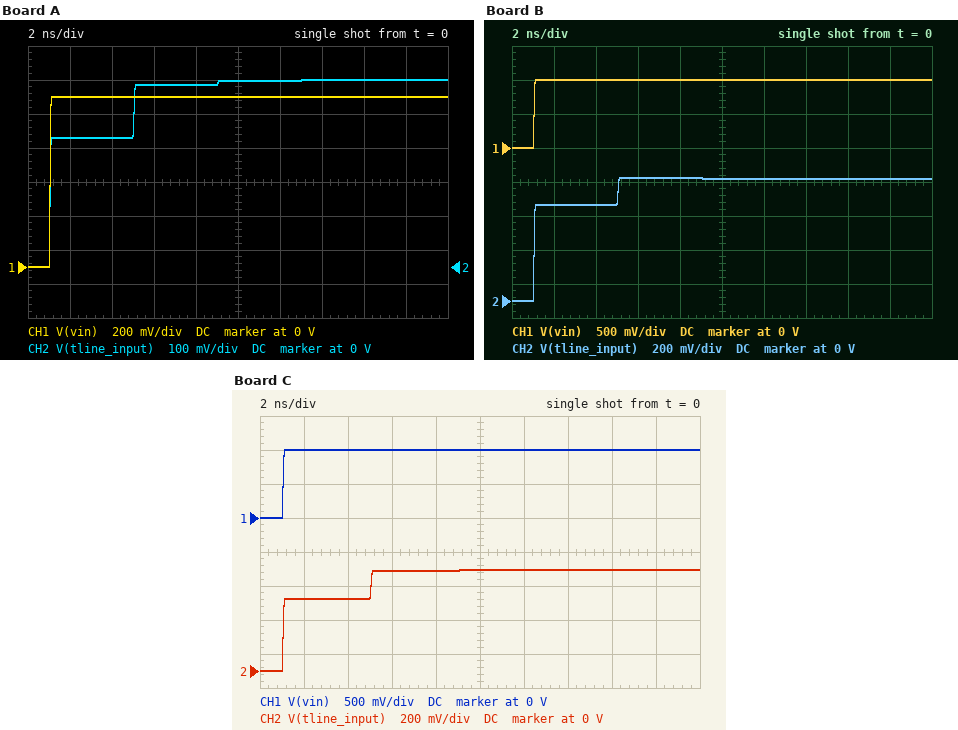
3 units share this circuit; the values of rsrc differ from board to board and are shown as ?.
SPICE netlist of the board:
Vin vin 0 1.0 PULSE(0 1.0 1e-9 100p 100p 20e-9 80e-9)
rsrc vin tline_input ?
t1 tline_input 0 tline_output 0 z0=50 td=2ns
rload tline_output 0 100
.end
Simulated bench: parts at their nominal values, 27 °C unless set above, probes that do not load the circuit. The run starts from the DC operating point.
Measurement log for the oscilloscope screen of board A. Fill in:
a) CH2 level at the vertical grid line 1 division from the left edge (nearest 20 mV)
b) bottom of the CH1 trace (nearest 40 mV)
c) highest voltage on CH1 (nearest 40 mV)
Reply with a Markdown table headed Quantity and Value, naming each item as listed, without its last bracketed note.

| Quantity | Value |
|---|---|
| CH2 level at the vertical grid line 1 division from the left edge | 380 mV |
| bottom of the CH1 trace | 0 V |
| highest voltage on CH1 | 1.00 V |
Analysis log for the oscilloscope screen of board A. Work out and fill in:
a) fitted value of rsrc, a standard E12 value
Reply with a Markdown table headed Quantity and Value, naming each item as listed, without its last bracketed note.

| Quantity | Value |
|---|---|
| fitted value of rsrc, a standard E12 value | 82 Ω |
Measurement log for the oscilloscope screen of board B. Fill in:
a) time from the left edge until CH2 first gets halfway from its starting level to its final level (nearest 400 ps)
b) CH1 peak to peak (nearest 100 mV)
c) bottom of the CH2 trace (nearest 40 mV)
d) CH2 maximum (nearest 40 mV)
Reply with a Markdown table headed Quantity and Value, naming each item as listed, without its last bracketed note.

| Quantity | Value |
|---|---|
| time from the left edge until CH2 first gets halfway from its starting level to its final level | 1.2 ns |
| CH1 peak to peak | 1.0 V |
| bottom of the CH2 trace | 0 V |
| CH2 maximum | 720 mV |
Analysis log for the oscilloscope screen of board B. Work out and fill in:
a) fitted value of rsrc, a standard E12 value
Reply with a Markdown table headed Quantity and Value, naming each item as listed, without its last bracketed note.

| Quantity | Value |
|---|---|
| fitted value of rsrc, a standard E12 value | 39 Ω |
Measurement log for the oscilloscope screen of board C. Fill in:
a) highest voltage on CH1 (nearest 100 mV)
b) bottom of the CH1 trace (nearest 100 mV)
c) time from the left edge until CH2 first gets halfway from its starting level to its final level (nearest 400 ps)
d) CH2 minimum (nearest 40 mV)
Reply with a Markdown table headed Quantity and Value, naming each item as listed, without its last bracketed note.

| Quantity | Value |
|---|---|
| highest voltage on CH1 | 1.0 V |
| bottom of the CH1 trace | 0 V |
| time from the left edge until CH2 first gets halfway from its starting level to its final level | 1.2 ns |
| CH2 minimum | 0 V |
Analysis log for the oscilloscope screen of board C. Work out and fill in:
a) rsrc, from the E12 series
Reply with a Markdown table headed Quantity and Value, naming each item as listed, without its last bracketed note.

| Quantity | Value |
|---|---|
| rsrc, from the E12 series | 68 Ω |
